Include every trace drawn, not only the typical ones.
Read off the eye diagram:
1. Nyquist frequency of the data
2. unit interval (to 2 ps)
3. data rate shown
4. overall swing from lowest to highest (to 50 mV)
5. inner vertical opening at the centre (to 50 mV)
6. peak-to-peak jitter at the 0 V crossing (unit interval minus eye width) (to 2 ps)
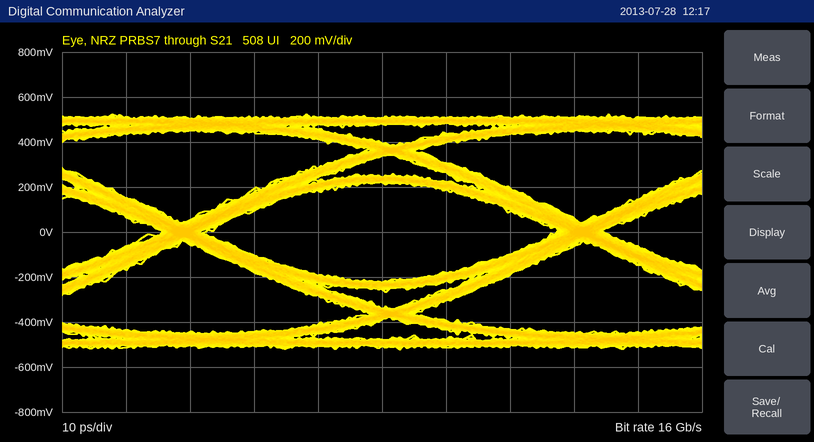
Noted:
8 GHz
62 ps
16 Gb/s
1.05 V
450 mV
8 ps
